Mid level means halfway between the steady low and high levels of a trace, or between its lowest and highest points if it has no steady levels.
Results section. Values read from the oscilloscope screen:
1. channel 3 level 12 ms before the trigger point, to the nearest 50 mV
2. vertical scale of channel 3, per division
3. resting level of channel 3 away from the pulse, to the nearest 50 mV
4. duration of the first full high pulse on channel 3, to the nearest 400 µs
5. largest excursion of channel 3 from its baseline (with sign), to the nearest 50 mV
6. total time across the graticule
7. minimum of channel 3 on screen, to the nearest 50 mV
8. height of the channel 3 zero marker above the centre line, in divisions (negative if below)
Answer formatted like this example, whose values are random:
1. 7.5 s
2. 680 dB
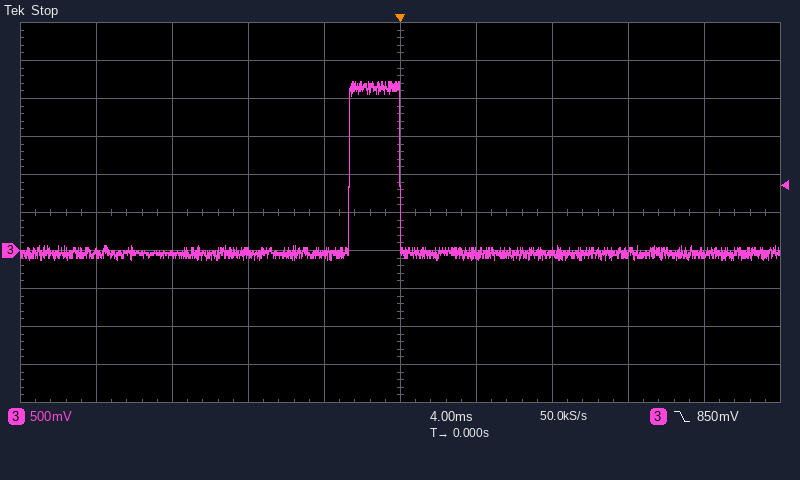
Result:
1. -50 mV
2. 500 mV
3. -50 mV
4. 2.8 ms
5. +2.25 V
6. 40 ms
7. -100 mV
8. -1.0 div
